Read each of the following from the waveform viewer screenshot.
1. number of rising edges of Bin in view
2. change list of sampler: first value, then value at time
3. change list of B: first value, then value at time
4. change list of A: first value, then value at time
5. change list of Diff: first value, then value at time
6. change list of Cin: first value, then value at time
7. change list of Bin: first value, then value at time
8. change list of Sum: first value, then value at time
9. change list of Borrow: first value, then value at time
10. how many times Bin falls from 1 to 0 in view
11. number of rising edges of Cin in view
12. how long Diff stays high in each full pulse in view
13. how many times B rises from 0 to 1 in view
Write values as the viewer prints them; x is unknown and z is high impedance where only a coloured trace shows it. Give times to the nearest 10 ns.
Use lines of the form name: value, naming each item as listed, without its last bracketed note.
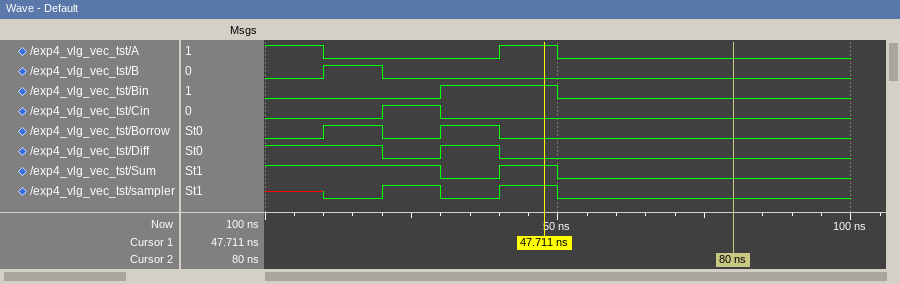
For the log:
number of rising edges of Bin in view: 1
change list of sampler: first value, then value at time: x, 0 at 10 ns, 1 at 20 ns, 0 at 30 ns, 1 at 40 ns, 0 at 50 ns
change list of B: first value, then value at time: 0, 1 at 10 ns, 0 at 20 ns
change list of A: first value, then value at time: 1, 0 at 10 ns, 1 at 40 ns, 0 at 50 ns
change list of Diff: first value, then value at time: 1, 0 at 20 ns, 1 at 30 ns, 0 at 40 ns
change list of Cin: first value, then value at time: 0, 1 at 20 ns, 0 at 30 ns
change list of Bin: first value, then value at time: 0, 1 at 30 ns, 0 at 50 ns
change list of Sum: first value, then value at time: 1, 0 at 30 ns, 1 at 40 ns, 0 at 50 ns
change list of Borrow: first value, then value at time: 0, 1 at 10 ns, 0 at 20 ns, 1 at 30 ns, 0 at 40 ns
how many times Bin falls from 1 to 0 in view: 1
number of rising edges of Cin in view: 1
how long Diff stays high in each full pulse in view: 10 ns
how many times B rises from 0 to 1 in view: 1
